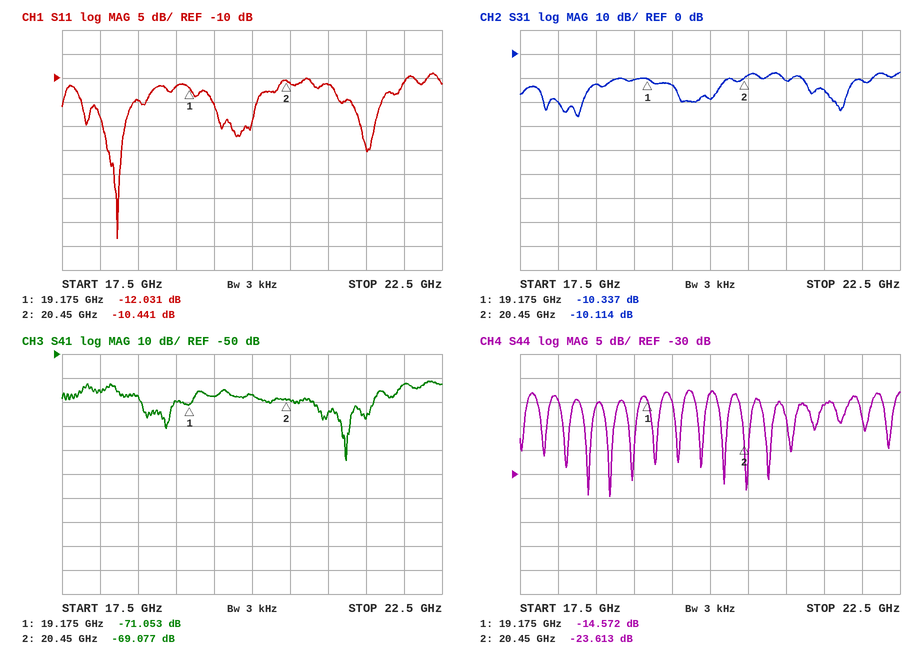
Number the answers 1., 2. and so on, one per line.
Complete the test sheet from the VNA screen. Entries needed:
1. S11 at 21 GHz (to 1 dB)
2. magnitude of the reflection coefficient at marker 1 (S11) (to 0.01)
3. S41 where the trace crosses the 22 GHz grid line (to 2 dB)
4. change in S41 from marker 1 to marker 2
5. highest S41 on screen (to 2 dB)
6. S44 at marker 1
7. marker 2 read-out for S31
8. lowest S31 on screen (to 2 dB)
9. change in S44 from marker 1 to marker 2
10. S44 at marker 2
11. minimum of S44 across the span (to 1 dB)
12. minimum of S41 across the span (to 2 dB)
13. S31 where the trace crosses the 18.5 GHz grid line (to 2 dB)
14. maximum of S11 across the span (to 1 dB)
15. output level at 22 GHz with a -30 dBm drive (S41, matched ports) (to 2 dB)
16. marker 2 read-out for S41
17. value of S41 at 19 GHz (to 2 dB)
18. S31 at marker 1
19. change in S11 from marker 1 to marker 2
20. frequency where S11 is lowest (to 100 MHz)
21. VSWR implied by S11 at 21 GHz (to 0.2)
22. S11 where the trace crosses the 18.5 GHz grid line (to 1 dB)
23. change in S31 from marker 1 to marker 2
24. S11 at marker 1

1. -11 dB
2. 0.25
3. -62 dB
4. 1.976 dB
5. -62 dB
6. -14.572 dB
7. -10.114 dB
8. -26 dB
9. -9.041 dB
10. -23.613 dB
11. -35 dB
12. -94 dB
13. -12 dB
14. -9 dB
15. -92 dBm
16. -69.077 dB
17. -70 dB
18. -10.337 dB
19. 1.590 dB
20. 18.2 GHz
21. 1.8
22. -15 dB
23. 0.223 dB
24. -12.031 dB
